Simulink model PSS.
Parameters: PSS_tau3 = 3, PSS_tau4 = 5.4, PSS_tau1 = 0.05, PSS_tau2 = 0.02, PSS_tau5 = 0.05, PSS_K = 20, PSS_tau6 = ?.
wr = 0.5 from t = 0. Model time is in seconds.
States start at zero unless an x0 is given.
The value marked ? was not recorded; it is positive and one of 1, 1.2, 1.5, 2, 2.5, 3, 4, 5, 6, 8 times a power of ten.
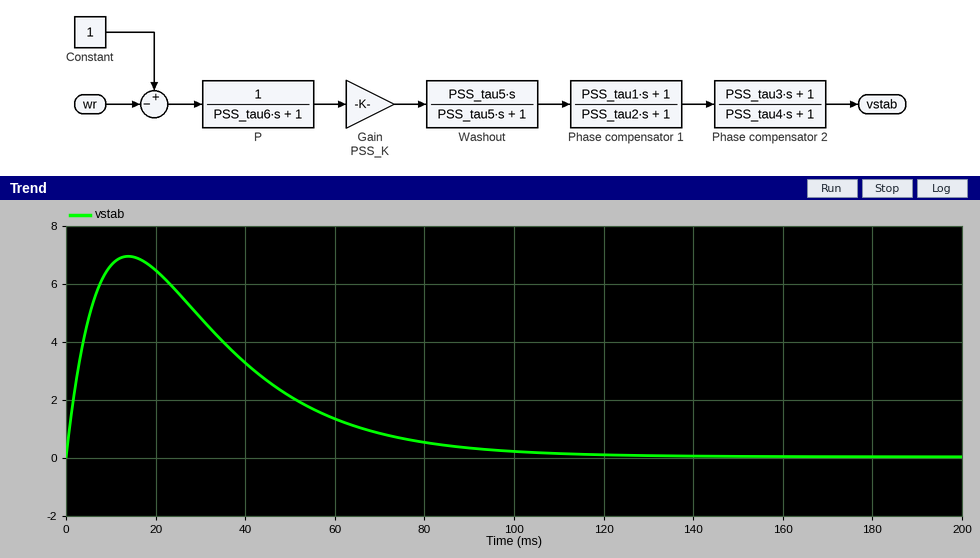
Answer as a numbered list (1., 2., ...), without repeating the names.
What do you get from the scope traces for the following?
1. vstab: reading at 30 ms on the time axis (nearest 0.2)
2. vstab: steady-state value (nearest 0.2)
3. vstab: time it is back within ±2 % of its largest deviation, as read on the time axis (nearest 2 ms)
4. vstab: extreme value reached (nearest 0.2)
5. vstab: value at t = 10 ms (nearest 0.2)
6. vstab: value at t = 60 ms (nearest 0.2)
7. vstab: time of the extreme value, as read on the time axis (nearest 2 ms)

1. 4.8
2. 0.0
3. 106 ms
4. 7.0
5. 6.6
6. 1.4
7. 14 ms
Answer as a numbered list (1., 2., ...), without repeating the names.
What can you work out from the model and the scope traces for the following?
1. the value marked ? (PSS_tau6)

1. 0.01
